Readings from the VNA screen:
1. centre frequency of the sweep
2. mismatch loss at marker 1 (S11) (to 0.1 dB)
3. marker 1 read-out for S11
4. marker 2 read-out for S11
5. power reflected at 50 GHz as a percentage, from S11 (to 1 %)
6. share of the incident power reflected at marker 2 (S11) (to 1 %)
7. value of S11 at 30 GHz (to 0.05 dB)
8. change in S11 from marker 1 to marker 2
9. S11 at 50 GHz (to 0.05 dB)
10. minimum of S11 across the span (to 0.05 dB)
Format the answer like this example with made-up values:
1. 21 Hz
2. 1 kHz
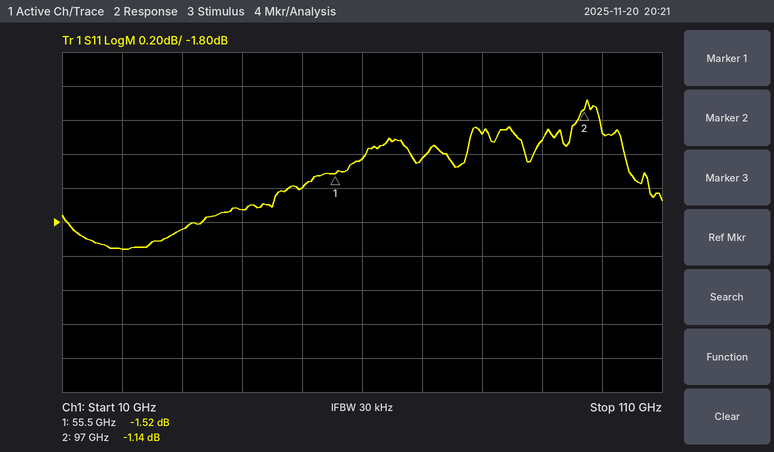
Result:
1. 60 GHz
2. 5.3 dB
3. -1.52 dB
4. -1.14 dB
5. 69 %
6. 77 %
7. -1.85 dB
8. 0.38 dB
9. -1.60 dB
10. -1.95 dB
